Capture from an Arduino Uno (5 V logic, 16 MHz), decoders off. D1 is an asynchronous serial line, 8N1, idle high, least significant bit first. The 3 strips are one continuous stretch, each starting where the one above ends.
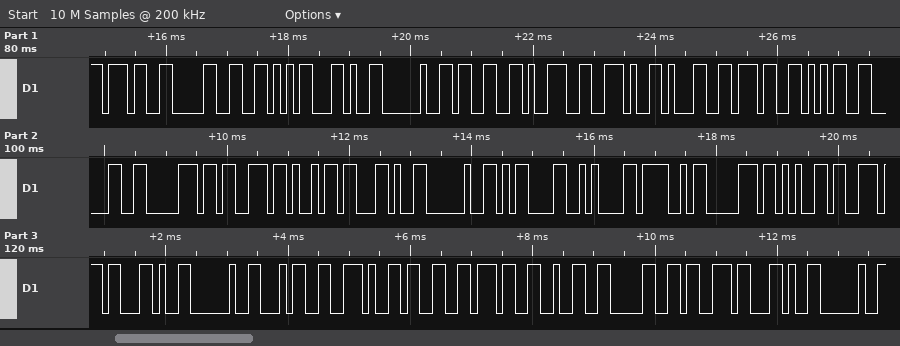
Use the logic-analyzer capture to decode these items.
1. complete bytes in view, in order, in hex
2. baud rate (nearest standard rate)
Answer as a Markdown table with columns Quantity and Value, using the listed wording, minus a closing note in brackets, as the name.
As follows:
| Quantity | Value |
|---|---|
| complete bytes in view, in order, in hex | 37 30 56 2C 20 33 39 2E 31 37 35 30 70 73 69 2C 20 0D 0A 4F 70 65 6E 2C 20 34 2E 33 37 32 30 73 2C 20 |
| baud rate | 9600 baud |
